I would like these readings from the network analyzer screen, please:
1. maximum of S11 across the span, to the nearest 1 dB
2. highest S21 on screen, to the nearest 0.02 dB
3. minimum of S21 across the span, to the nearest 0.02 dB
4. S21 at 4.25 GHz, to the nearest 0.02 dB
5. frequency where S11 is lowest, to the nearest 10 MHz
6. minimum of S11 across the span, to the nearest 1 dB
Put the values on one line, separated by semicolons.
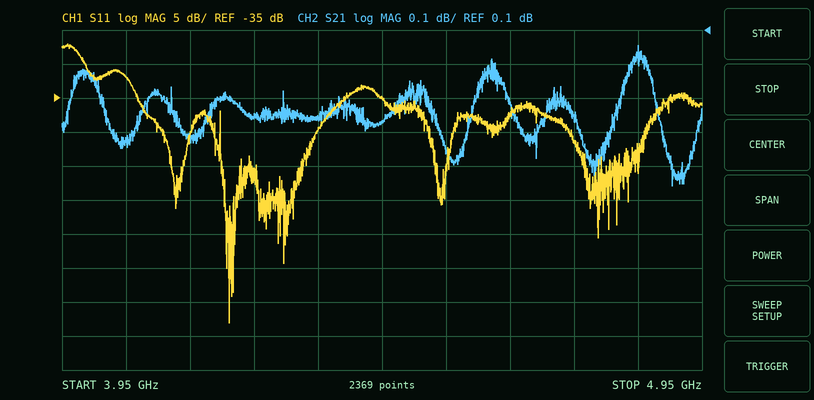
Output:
-27 dB; 0.06 dB; -0.36 dB; -0.16 dB; 4.21 GHz; -68 dB
